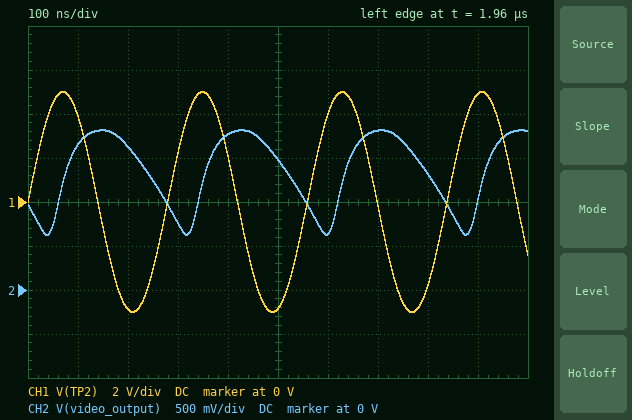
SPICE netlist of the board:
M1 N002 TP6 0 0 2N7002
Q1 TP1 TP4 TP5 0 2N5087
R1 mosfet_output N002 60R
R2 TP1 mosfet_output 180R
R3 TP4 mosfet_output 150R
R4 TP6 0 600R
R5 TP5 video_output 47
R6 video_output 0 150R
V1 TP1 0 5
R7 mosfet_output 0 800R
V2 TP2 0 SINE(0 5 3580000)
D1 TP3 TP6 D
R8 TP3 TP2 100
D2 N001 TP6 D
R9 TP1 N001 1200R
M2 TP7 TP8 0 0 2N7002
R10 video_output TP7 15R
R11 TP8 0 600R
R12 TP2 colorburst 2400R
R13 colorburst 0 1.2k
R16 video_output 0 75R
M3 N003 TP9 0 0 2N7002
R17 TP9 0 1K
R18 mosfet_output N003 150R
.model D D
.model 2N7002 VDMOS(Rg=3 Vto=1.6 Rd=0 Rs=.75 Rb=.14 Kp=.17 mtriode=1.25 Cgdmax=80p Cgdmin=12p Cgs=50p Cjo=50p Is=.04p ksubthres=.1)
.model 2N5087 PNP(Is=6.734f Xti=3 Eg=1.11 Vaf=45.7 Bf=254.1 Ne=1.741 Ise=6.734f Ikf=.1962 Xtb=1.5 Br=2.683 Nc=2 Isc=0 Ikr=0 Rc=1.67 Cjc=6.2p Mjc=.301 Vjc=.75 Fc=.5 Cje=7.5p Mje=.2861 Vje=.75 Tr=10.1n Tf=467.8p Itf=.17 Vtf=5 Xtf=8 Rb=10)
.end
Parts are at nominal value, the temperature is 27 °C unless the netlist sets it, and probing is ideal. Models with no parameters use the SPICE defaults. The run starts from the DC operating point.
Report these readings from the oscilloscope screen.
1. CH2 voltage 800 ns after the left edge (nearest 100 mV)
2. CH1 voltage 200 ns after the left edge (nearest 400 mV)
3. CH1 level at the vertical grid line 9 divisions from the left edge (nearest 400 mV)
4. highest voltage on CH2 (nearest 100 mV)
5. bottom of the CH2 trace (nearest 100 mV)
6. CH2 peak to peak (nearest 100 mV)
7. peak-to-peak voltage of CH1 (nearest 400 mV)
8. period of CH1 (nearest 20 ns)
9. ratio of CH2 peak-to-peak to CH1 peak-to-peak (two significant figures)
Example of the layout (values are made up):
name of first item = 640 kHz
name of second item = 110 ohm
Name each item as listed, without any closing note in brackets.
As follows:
CH2 voltage 800 ns after the left edge = 1.3 V
CH1 voltage 200 ns after the left edge = -4.8 V
CH1 level at the vertical grid line 9 divisions from the left edge = 4.8 V
highest voltage on CH2 = 1.8 V
bottom of the CH2 trace = 600 mV
CH2 peak to peak = 1.2 V
peak-to-peak voltage of CH1 = 10.0 V
period of CH1 = 280 ns
ratio of CH2 peak-to-peak to CH1 peak-to-peak = 0.12
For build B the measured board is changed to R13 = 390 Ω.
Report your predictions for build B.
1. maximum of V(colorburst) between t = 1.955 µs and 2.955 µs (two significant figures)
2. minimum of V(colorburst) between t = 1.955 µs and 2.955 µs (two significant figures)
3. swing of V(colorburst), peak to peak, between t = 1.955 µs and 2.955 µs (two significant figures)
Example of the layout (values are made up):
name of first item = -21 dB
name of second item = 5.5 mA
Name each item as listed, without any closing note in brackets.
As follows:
maximum of V(colorburst) between t = 1.955 µs and 2.955 µs = 700 mV
minimum of V(colorburst) between t = 1.955 µs and 2.955 µs = -700 mV
swing of V(colorburst), peak to peak, between t = 1.955 µs and 2.955 µs = 1.4 V
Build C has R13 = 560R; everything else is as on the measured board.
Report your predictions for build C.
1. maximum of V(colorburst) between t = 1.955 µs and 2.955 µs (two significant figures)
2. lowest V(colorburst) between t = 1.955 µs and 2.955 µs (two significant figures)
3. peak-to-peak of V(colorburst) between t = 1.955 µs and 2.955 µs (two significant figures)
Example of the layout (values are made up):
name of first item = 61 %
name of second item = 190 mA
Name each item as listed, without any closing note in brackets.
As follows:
maximum of V(colorburst) between t = 1.955 µs and 2.955 µs = 950 mV
lowest V(colorburst) between t = 1.955 µs and 2.955 µs = -950 mV
peak-to-peak of V(colorburst) between t = 1.955 µs and 2.955 µs = 1.9 V
